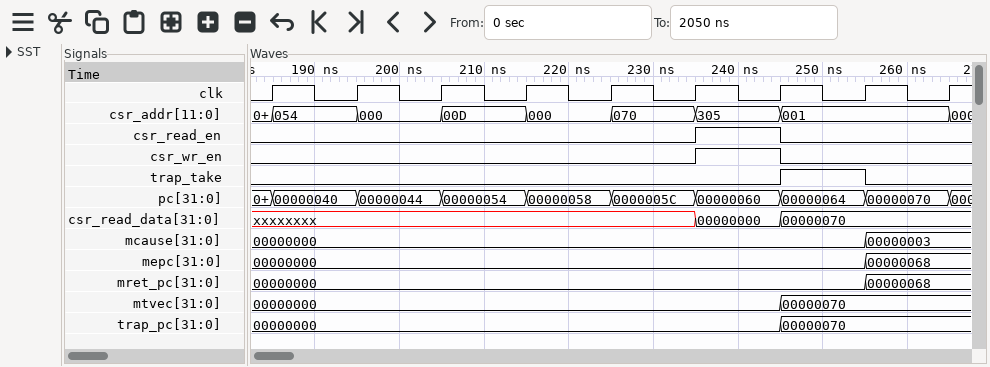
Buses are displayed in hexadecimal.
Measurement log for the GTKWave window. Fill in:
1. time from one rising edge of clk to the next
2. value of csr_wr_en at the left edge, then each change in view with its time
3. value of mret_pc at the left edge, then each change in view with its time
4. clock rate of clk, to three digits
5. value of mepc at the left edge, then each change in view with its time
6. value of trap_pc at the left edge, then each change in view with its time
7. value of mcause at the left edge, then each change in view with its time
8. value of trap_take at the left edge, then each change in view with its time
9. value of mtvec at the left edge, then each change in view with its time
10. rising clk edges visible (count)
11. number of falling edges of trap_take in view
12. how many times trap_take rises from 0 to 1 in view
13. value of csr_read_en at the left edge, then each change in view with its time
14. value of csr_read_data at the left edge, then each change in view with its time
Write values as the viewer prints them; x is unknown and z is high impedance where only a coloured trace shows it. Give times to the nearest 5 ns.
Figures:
10 ns
0, 1 at 235 ns, 0 at 245 ns
00000000, 00000068 at 255 ns
100 MHz
00000000, 00000068 at 255 ns
00000000, 00000070 at 245 ns
00000000, 00000003 at 255 ns
0, 1 at 245 ns, 0 at 255 ns
00000000, 00000070 at 245 ns
9
1
1
0, 1 at 235 ns, 0 at 245 ns
xxxxxxxx, 00000000 at 235 ns, 00000070 at 245 ns
